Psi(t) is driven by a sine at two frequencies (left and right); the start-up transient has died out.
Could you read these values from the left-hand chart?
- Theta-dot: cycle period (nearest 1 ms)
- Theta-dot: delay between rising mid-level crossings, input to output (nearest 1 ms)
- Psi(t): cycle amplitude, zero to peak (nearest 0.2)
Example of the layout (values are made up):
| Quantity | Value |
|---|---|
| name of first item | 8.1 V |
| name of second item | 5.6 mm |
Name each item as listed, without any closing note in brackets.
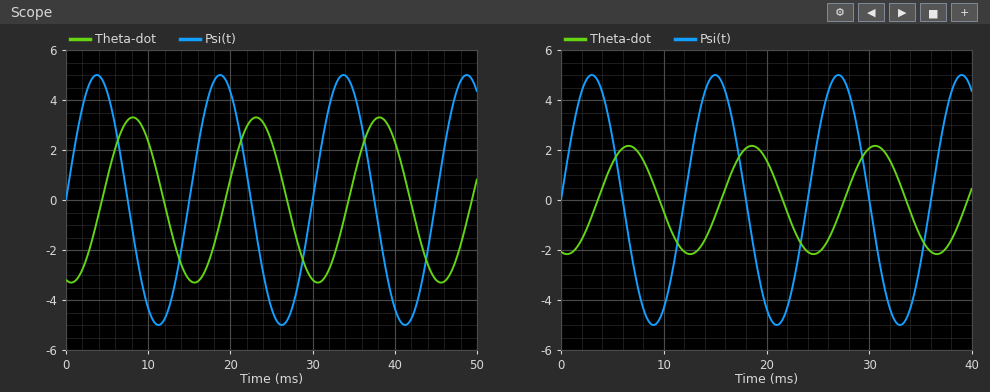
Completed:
| Quantity | Value |
|---|---|
| Theta-dot: cycle period | 15 ms |
| Theta-dot: delay between rising mid-level crossings, input to output | 4 ms |
| Psi(t): cycle amplitude, zero to peak | 5.0 |
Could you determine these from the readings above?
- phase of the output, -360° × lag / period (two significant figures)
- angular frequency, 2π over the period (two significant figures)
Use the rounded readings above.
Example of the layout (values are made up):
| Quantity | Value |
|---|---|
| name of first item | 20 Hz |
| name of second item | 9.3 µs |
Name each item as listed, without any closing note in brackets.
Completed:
| Quantity | Value |
|---|---|
| phase of the output, -360° × lag / period | -96° |
| angular frequency, 2π over the period | 0.42 rad/ms |
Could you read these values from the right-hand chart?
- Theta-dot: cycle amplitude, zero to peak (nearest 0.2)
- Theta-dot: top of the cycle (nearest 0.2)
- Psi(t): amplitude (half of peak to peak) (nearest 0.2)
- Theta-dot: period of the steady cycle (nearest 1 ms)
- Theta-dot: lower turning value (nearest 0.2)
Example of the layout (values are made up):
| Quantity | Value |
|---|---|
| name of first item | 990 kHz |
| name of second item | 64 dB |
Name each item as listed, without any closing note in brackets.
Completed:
| Quantity | Value |
|---|---|
| Theta-dot: cycle amplitude, zero to peak | 2.2 |
| Theta-dot: top of the cycle | 2.2 |
| Psi(t): amplitude (half of peak to peak) | 5.0 |
| Theta-dot: period of the steady cycle | 12 ms |
| Theta-dot: lower turning value | -2.2 |
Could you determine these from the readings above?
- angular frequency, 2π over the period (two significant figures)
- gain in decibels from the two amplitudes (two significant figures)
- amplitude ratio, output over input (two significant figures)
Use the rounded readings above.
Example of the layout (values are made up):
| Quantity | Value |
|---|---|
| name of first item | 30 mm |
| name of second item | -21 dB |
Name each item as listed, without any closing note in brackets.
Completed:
| Quantity | Value |
|---|---|
| angular frequency, 2π over the period | 0.52 rad/ms |
| gain in decibels from the two amplitudes | -7.1 dB |
| amplitude ratio, output over input | 0.44 |
